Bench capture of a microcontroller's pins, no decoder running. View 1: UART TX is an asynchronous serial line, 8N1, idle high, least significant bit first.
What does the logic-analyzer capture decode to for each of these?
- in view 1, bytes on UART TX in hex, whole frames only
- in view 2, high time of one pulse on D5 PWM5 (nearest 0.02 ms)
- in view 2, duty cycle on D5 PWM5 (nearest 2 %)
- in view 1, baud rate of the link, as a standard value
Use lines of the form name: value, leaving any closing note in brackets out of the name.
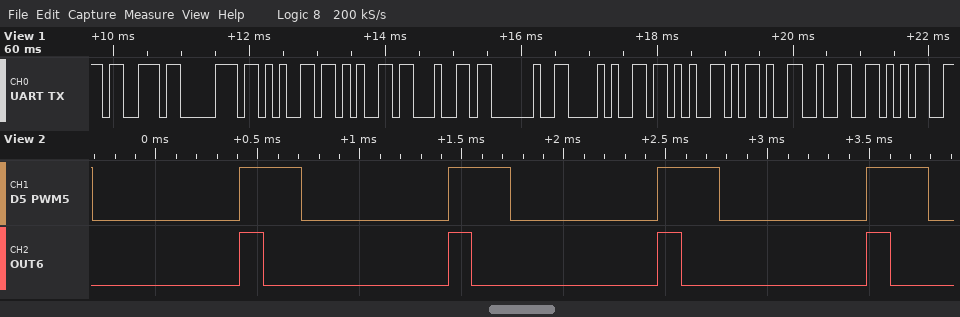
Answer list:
in view 1, bytes on UART TX in hex, whole frames only: 73 70 65 65 64 20 28 2B 2D 32 35
in view 2, high time of one pulse on D5 PWM5: 0.30 ms
in view 2, duty cycle on D5 PWM5: 30 %
in view 1, baud rate of the link, as a standard value: 9600 baud
